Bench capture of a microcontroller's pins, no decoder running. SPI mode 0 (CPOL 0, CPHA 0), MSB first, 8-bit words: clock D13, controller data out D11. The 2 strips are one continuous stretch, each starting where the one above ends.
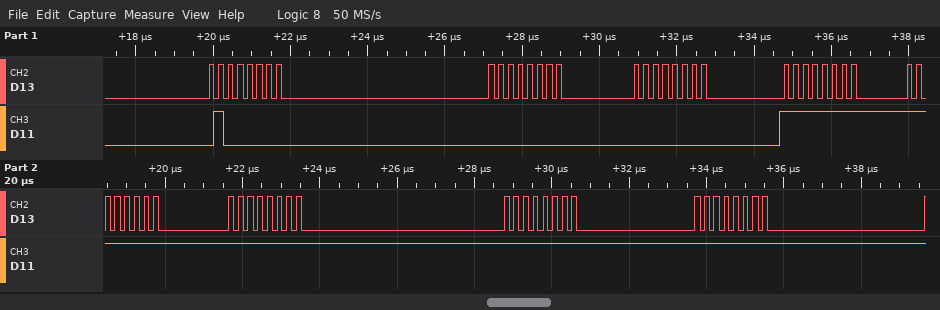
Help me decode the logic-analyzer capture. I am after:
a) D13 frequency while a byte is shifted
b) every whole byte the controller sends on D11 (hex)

4 MHz
40 00 00 FF FF FF FF FF
